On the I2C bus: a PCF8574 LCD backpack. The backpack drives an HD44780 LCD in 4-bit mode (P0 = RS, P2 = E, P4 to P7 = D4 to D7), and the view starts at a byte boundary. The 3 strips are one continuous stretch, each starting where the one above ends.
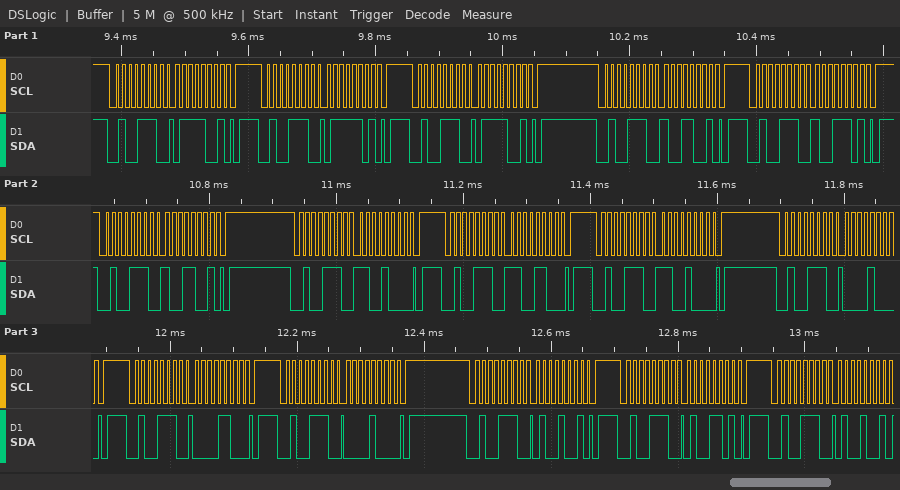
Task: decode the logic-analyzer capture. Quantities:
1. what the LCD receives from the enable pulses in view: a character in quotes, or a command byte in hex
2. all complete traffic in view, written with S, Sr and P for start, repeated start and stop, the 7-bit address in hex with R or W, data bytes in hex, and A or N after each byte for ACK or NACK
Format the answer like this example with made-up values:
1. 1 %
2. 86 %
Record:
1. 'y' 0xC0
2. S 27W A 79 A P S 27W A 7D A P S 27W A 79 A P S 27W A 99 A P S 27W A 9D A P S 27W A 99 A P S 27W A C8 A P S 27W A CC A P S 27W A C8 A P S 27W A 08 A P S 27W A 0C A P S 27W A 08 A P S 27W A 49 A P S 27W A 4D A P S 27W A 49 A
